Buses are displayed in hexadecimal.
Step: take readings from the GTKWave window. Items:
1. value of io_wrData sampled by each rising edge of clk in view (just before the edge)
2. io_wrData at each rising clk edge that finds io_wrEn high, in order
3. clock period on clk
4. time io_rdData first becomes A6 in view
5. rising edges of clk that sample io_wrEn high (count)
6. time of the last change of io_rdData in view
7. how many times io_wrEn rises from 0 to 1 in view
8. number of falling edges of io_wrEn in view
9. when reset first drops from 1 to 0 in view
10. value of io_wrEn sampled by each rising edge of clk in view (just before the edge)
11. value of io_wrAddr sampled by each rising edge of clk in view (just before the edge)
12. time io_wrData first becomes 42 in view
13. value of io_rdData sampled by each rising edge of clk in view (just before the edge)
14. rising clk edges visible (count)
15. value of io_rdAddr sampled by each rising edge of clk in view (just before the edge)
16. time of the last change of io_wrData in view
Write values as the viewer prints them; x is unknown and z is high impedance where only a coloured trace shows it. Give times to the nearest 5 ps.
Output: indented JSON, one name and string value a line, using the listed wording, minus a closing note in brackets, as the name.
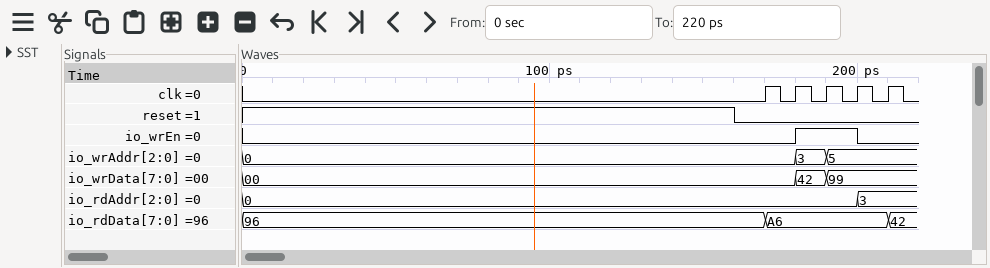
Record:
{
  "value of io_wrData sampled by each rising edge of clk in view": "00, 00, 42, 99, 99",
  "io_wrData at each rising clk edge that finds io_wrEn high, in order": "42, 99",
  "clock period on clk": "10 ps",
  "time io_rdData first becomes A6 in view": "170 ps",
  "rising edges of clk that sample io_wrEn high": "2",
  "time of the last change of io_rdData in view": "210 ps",
  "how many times io_wrEn rises from 0 to 1 in view": "1",
  "number of falling edges of io_wrEn in view": "1",
  "when reset first drops from 1 to 0 in view": "160 ps",
  "value of io_wrEn sampled by each rising edge of clk in view": "0 0 1 1 0",
  "value of io_wrAddr sampled by each rising edge of clk in view": "0, 0, 3, 5, 5",
  "time io_wrData first becomes 42 in view": "180 ps",
  "value of io_rdData sampled by each rising edge of clk in view": "96, A6, A6, A6, A6",
  "rising clk edges visible": "5",
  "value of io_rdAddr sampled by each rising edge of clk in view": "0, 0, 0, 0, 3",
  "time of the last change of io_wrData in view": "190 ps"
}
